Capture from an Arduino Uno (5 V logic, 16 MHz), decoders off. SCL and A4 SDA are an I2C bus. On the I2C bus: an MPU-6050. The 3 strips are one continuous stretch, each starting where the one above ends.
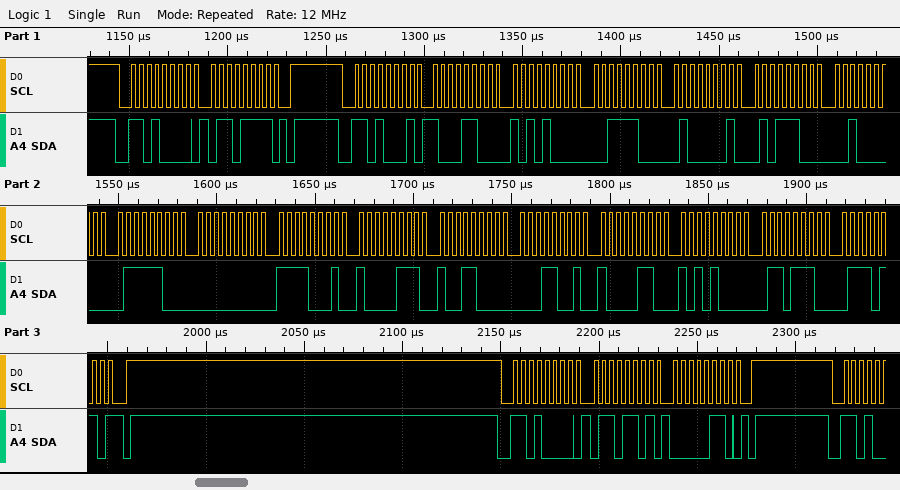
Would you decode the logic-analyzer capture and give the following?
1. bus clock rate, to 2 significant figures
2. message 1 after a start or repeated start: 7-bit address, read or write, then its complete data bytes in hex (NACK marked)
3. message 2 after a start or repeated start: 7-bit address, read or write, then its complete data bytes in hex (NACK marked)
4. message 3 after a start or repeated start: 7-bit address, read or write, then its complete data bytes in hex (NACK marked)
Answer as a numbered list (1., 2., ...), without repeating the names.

1. 250 kHz
2. 0x68 write: 6F
3. 0x68 read: 8C A8 3C 41 5C 20 7C 00 F1 87 98 19 86 A8 6E 76 NACK
4. 0x68 write: 6D 06
